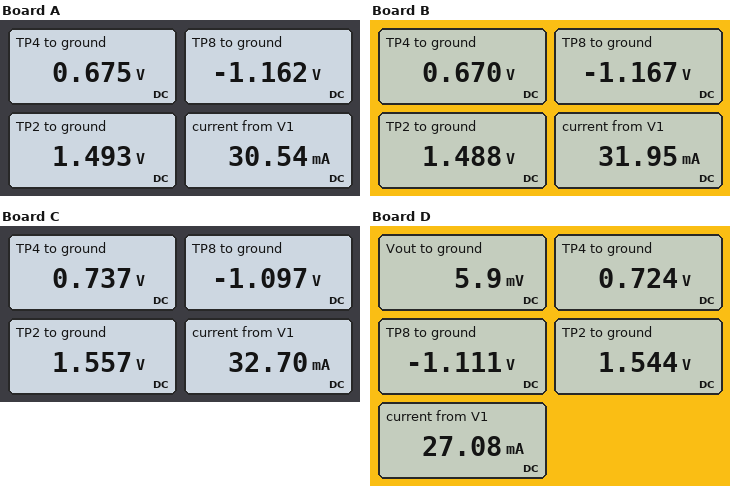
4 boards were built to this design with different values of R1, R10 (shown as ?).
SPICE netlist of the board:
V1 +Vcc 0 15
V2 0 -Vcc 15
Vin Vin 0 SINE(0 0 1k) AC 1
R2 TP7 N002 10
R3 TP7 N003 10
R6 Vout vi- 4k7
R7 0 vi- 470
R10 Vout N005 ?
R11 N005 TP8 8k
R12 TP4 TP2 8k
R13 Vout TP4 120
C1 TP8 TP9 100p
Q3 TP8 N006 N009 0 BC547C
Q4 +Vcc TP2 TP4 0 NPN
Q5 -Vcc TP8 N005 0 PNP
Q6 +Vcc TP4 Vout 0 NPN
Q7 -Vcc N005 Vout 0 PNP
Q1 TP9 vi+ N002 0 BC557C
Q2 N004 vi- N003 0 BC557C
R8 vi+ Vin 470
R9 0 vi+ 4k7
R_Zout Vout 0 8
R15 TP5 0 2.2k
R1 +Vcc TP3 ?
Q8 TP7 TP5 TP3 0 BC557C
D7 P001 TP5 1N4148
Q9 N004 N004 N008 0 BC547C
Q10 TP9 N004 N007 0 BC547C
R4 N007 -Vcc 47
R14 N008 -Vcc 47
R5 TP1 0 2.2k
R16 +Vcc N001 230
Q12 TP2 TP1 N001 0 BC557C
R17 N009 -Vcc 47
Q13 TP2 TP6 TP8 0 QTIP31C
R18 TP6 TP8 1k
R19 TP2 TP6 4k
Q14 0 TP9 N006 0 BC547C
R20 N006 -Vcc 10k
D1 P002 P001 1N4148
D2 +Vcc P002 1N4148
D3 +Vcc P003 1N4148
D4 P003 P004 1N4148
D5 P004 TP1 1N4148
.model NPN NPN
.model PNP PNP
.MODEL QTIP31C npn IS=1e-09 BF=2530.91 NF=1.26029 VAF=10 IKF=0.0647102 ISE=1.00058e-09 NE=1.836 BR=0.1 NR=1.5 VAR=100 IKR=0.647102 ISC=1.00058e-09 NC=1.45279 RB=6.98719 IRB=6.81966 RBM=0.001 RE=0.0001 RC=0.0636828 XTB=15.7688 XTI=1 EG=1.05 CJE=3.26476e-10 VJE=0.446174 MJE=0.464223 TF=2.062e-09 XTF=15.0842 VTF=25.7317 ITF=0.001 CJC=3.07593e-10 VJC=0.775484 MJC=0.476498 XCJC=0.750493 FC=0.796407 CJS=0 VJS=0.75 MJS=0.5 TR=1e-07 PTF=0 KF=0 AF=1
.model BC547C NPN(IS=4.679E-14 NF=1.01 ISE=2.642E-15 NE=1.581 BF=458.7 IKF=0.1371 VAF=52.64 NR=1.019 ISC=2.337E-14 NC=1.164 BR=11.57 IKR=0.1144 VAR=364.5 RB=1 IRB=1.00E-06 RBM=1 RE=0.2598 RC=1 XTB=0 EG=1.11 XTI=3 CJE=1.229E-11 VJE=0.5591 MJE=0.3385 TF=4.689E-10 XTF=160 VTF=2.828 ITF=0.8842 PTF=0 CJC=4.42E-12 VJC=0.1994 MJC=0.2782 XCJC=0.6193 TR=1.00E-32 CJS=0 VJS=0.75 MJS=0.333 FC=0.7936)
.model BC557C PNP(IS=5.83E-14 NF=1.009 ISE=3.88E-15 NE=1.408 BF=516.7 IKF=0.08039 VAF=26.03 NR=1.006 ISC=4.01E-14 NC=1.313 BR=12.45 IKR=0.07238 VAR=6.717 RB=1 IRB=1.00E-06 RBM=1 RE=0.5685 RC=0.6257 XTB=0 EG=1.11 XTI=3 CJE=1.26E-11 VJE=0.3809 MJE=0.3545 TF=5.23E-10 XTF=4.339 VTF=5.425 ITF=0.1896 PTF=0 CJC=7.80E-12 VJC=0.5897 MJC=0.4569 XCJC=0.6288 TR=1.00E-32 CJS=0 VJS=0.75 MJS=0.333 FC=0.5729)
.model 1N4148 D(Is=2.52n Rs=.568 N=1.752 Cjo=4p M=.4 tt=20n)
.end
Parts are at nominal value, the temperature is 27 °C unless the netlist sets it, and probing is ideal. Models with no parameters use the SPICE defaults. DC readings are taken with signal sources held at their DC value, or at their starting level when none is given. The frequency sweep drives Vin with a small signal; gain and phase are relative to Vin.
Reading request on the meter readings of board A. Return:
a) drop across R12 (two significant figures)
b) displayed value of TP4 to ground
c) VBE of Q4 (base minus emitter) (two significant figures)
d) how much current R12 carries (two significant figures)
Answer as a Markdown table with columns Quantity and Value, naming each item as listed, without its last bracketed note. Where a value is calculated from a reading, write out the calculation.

| Quantity | Value |
|---|---|
| drop across R12 | 1.493 V - 675 mV = 820 mV |
| displayed value of TP4 to ground | 0.675 V |
| VBE of Q4 (base minus emitter) | 1.493 V - 675 mV = 820 mV |
| how much current R12 carries | (1.493 V - 675 mV) / 8 kΩ = 100 µA |
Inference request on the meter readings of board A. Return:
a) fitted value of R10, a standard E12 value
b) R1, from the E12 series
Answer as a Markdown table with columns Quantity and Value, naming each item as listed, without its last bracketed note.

| Quantity | Value |
|---|---|
| fitted value of R10, a standard E12 value | 68 Ω |
| R1, from the E12 series | 180 Ω |
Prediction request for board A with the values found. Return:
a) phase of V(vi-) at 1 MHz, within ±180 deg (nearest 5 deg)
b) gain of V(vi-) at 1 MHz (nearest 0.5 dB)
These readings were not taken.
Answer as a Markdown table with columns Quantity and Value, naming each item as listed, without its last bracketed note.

| Quantity | Value |
|---|---|
| phase of V(vi-) at 1 MHz, within ±180 deg | -45 deg |
| gain of V(vi-) at 1 MHz | -3.0 dB |
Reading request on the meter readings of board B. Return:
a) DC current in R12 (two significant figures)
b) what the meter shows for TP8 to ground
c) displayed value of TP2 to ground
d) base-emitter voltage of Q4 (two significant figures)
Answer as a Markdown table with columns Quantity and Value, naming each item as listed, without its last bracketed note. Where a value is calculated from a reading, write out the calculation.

| Quantity | Value |
|---|---|
| DC current in R12 | (1.488 V - 670 mV) / 8 kΩ = 100 µA |
| what the meter shows for TP8 to ground | -1.167 V |
| displayed value of TP2 to ground | 1.488 V |
| base-emitter voltage of Q4 | 1.488 V - 670 mV = 820 mV |
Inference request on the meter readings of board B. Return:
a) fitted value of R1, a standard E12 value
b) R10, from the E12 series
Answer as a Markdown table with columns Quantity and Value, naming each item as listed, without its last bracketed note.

| Quantity | Value |
|---|---|
| fitted value of R1, a standard E12 value | 150 Ω |
| R10, from the E12 series | 68 Ω |
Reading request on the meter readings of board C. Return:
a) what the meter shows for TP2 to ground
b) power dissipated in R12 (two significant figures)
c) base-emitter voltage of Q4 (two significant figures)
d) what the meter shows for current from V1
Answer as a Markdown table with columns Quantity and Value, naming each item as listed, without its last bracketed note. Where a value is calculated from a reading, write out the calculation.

| Quantity | Value |
|---|---|
| what the meter shows for TP2 to ground | 1.557 V |
| power dissipated in R12 | (1.557 V - 737 mV)^2 / 8 kΩ = 84 µW |
| base-emitter voltage of Q4 | 1.557 V - 737 mV = 820 mV |
| what the meter shows for current from V1 | 32.70 mA |
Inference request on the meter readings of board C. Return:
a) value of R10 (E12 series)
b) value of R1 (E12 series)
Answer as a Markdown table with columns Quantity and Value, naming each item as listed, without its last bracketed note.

| Quantity | Value |
|---|---|
| value of R10 | 47 Ω |
| value of R1 | 150 Ω |
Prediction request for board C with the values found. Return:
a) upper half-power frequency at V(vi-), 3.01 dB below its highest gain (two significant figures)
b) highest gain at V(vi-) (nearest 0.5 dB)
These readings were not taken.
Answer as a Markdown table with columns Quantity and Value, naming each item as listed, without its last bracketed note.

| Quantity | Value |
|---|---|
| upper half-power frequency at V(vi-), 3.01 dB below its highest gain | 2.0 MHz |
| highest gain at V(vi-) | -1.0 dB |
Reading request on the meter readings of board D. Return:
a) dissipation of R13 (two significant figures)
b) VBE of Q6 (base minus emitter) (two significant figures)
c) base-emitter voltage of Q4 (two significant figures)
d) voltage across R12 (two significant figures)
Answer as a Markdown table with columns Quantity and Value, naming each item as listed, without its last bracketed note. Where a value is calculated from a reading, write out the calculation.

| Quantity | Value |
|---|---|
| dissipation of R13 | (724 mV - 5.9 mV)^2 / 120 Ω = 4.3 mW |
| VBE of Q6 (base minus emitter) | 724 mV - 5.9 mV = 720 mV |
| base-emitter voltage of Q4 | 1.544 V - 724 mV = 820 mV |
| voltage across R12 | 1.544 V - 724 mV = 820 mV |
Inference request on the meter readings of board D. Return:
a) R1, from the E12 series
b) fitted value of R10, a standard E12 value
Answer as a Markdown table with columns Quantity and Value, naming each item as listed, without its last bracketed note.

| Quantity | Value |
|---|---|
| R1, from the E12 series | 390 Ω |
| fitted value of R10, a standard E12 value | 56 Ω |
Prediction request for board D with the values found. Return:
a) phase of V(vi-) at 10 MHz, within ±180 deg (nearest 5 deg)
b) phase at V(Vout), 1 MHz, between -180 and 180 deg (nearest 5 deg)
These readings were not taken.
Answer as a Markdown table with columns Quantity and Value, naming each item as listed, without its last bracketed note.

| Quantity | Value |
|---|---|
| phase of V(vi-) at 10 MHz, within ±180 deg | 40 deg |
| phase at V(Vout), 1 MHz, between -180 and 180 deg | -50 deg |
